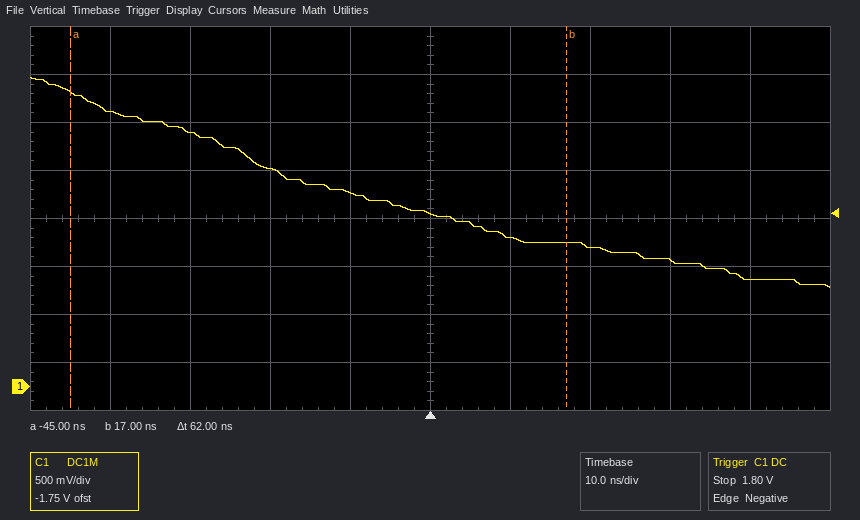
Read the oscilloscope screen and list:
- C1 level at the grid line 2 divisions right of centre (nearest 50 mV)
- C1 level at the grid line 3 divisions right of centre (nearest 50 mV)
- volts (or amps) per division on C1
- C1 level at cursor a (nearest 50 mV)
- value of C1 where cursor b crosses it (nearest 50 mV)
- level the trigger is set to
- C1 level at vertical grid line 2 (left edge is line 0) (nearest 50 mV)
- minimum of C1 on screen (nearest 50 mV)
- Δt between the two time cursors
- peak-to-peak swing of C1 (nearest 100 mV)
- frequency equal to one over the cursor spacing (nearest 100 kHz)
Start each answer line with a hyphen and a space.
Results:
- 1.45 V
- 1.30 V
- 500 mV
- 3.05 V
- 1.50 V
- 1.80 V
- 2.65 V
- 1.05 V
- 62 ns
- 2.20 V
- 16.1 MHz
